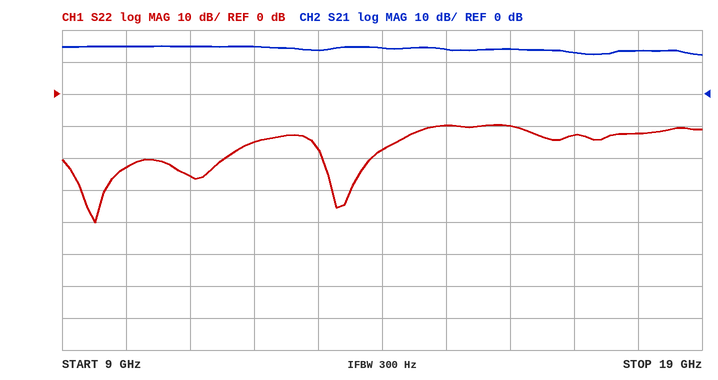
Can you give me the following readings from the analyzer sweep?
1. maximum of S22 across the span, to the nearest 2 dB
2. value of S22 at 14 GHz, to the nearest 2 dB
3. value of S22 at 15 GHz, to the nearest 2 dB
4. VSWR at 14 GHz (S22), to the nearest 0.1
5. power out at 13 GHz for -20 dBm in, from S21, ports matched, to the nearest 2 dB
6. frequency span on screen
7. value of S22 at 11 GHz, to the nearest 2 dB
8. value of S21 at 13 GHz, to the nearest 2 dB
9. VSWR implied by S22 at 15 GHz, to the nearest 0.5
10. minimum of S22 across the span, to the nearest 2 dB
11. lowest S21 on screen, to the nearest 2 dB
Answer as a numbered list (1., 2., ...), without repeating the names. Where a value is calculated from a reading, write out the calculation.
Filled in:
1. -10 dB
2. -18 dB
3. -10 dB
4. |Γ| = 10^(-18/20) = 0.1259; VSWR = (1 + 0.1259)/(1 − 0.1259) ≈ 1.3
5. -20 dBm + (14 dB) = -6 dBm
6. 10 GHz
7. -26 dB
8. 14 dB
9. |Γ| = 10^(-10/20) = 0.3162; VSWR = (1 + 0.3162)/(1 − 0.3162) ≈ 1.92, so 2.0 to the nearest 0.5
10. -40 dB
11. 12 dB
